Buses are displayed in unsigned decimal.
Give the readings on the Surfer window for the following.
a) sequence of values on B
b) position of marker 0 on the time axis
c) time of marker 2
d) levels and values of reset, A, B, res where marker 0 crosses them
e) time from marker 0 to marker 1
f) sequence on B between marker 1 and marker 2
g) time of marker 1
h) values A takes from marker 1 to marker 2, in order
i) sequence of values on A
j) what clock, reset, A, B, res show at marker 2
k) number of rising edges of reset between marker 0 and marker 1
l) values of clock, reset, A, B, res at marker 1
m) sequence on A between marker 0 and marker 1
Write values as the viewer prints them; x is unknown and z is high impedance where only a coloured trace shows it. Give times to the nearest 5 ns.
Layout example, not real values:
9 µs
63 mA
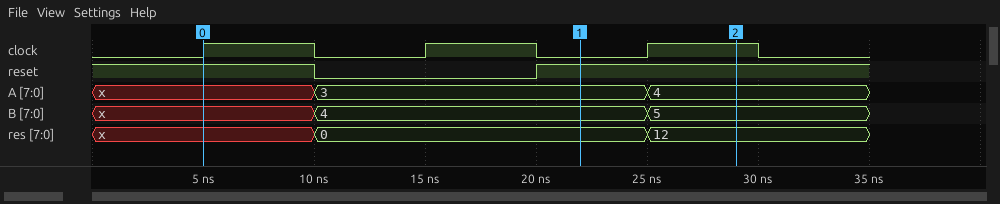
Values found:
x, 4, 5
5 ns
30 ns
reset=1, A=x, B=x, res=x
15 ns
4, 5
20 ns
3, 4
x, 3, 4
clock=1, reset=1, A=4, B=5, res=12
1
clock=0, reset=1, A=3, B=4, res=0
x, 3
